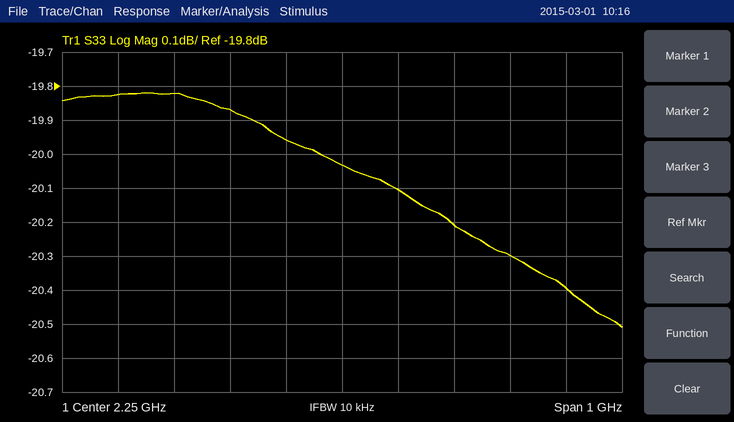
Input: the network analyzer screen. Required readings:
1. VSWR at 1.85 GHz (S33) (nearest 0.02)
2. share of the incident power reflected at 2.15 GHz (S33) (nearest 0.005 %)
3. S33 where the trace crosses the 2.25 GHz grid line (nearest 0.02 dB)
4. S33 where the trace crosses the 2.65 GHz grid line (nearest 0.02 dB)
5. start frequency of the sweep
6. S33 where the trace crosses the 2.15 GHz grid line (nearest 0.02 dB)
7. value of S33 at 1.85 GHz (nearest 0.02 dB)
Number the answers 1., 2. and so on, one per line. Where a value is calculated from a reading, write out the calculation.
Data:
1. |Γ| = 10^(-19.82/20) = 0.1021; VSWR = (1 + 0.1021)/(1 − 0.1021) ≈ 1.23, so 1.22 to the nearest 0.02
2. 10^(-19.96/10) ≈ 1.010 %
3. -20.04 dB
4. -20.40 dB
5. 1.75 GHz
6. -19.96 dB
7. -19.82 dB
